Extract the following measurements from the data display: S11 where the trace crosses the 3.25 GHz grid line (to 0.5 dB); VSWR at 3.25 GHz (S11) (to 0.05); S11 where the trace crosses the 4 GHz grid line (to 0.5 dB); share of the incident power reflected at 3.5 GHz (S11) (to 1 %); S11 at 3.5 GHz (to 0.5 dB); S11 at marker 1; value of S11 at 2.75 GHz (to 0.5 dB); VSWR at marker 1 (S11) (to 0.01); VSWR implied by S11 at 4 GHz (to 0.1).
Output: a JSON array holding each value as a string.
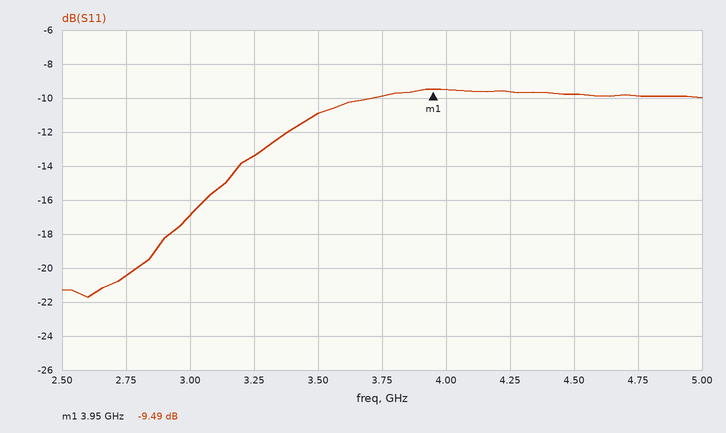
["-13.5 dB", "1.55", "-9.5 dB", "8 %", "-11.0 dB", "-9.49 dB", "-20.5 dB", "2.01", "2.0"]
